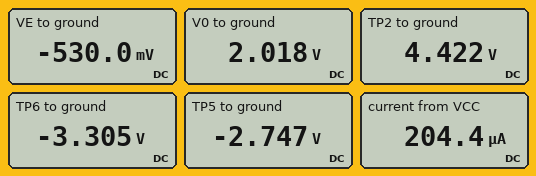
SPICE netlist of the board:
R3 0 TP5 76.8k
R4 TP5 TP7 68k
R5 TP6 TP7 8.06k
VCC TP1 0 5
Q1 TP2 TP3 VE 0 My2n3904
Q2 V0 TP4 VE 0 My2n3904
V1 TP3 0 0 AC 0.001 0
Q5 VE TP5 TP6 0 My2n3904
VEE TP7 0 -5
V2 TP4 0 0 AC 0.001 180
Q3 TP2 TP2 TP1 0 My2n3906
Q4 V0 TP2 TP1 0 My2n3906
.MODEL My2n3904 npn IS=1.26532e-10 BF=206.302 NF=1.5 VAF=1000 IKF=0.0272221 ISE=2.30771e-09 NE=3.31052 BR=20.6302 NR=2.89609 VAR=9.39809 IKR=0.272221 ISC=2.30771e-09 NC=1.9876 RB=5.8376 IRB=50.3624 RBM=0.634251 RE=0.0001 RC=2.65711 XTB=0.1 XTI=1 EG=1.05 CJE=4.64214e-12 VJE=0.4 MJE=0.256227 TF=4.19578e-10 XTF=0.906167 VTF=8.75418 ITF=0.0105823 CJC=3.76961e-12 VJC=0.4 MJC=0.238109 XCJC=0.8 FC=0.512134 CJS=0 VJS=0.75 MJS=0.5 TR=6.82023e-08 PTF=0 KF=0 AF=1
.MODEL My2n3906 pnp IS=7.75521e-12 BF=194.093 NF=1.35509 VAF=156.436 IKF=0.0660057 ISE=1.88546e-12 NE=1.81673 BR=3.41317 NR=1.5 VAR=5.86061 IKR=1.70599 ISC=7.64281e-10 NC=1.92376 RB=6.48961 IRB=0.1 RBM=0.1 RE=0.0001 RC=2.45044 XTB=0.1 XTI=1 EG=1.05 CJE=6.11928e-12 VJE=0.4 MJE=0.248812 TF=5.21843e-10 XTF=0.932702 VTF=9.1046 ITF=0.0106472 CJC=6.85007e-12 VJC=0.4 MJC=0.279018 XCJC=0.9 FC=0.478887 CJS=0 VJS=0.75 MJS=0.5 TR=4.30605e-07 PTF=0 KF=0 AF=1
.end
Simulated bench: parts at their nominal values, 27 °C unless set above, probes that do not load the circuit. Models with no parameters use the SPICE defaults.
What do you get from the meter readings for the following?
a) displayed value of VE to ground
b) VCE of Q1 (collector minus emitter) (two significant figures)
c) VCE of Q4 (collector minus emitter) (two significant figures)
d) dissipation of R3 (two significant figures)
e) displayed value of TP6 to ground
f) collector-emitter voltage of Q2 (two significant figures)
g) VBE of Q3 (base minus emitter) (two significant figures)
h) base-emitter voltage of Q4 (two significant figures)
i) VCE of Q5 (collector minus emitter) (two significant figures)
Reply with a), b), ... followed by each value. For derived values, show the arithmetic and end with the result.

a) -530.0 mV
b) 4.422 V - (-530 mV) = 5.0 V
c) 2.018 V - 5 V = -3.0 V
d) (0 V - (-2.747 V))^2 / 76.8 kΩ = 98 µW
e) -3.305 V
f) 2.018 V - (-530 mV) = 2.5 V
g) 4.422 V - 5 V = -580 mV
h) 4.422 V - 5 V = -580 mV
i) -530 mV - (-3.305 V) = 2.8 V
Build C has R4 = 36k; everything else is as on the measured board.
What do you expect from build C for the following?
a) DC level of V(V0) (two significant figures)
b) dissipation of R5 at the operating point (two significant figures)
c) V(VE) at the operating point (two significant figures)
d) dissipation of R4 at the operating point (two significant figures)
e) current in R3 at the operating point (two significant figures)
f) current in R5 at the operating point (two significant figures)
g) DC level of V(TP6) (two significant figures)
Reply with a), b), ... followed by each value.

a) 1.9 V
b) 130 µW
c) -510 mV
d) 67 µW
e) 45 µA
f) 130 µA
g) -4.0 V
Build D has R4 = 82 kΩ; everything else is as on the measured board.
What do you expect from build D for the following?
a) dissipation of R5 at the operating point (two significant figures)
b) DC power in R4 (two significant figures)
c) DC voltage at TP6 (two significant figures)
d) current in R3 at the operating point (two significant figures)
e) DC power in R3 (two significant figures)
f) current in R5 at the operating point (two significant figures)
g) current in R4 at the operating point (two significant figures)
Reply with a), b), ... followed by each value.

a) 450 µW
b) 74 µW
c) -3.1 V
d) 33 µA
e) 83 µW
f) 240 µA
g) 30 µA
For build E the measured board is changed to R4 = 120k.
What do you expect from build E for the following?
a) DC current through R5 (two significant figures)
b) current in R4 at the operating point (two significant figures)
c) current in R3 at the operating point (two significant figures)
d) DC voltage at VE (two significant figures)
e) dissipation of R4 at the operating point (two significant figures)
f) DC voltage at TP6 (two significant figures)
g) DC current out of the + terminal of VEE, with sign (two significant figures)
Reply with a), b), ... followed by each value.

a) 290 µA
b) 24 µA
c) 27 µA
d) -540 mV
e) 70 µW
f) -2.7 V
g) -310 µA
